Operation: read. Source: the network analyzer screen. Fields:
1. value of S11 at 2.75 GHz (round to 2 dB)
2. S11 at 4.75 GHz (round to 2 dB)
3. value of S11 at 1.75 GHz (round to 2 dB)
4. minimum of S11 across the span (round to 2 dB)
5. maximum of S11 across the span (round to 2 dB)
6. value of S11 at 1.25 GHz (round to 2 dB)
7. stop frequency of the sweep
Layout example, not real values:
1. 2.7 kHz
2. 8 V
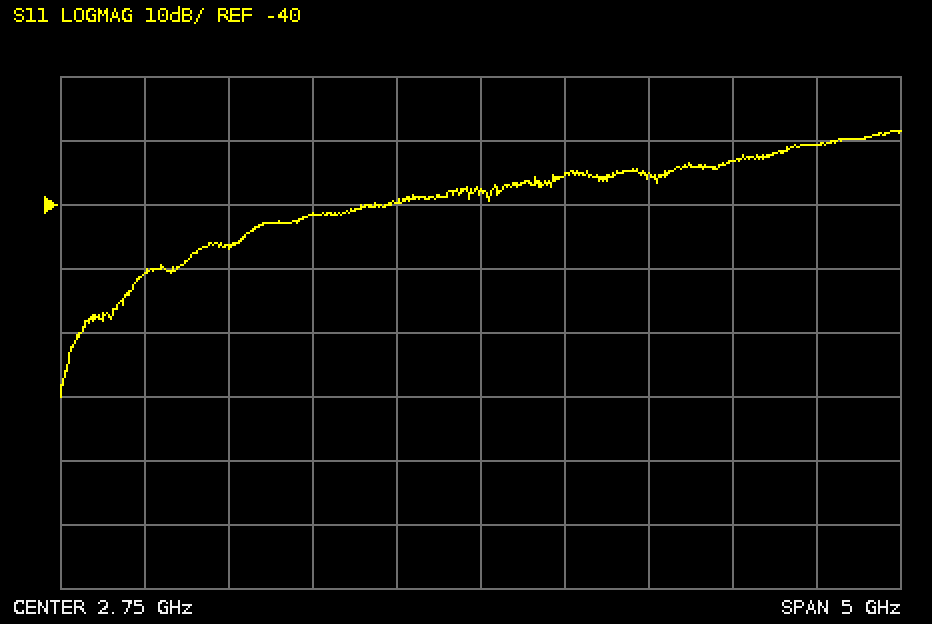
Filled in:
1. -38 dB
2. -30 dB
3. -42 dB
4. -70 dB
5. -28 dB
6. -46 dB
7. 5.25 GHz
